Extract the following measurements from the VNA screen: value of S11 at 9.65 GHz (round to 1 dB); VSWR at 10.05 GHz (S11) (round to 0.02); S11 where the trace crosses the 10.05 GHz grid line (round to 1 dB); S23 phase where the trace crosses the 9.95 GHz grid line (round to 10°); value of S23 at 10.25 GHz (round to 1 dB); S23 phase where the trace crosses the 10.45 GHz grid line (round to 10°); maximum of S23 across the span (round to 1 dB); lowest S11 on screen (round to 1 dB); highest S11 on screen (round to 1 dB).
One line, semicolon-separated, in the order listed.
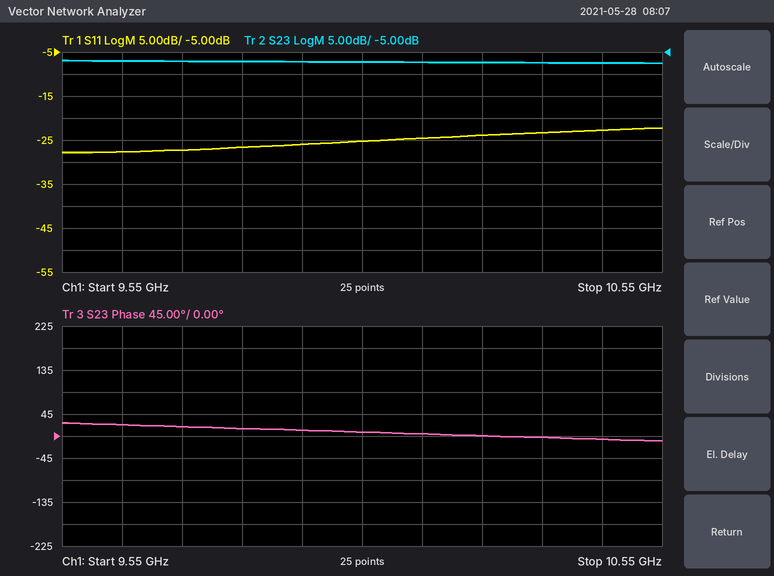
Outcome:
-28 dB; 1.12; -25 dB; 10°; -7 dB; -10°; -7 dB; -28 dB; -22 dB
